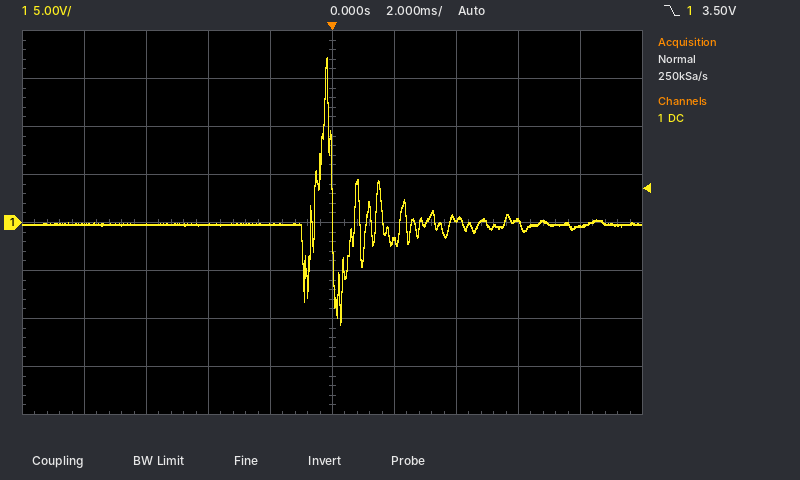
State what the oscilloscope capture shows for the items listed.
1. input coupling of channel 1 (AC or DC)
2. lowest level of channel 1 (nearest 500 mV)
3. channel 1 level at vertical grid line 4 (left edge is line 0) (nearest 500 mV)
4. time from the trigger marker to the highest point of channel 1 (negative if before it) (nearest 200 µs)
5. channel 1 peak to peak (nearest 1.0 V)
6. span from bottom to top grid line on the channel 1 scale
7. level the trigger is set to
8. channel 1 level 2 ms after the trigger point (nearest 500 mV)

DC
-10.5 V
0.0 V
-200 µs
28.0 V
40 V
3.50 V
-2.0 V
